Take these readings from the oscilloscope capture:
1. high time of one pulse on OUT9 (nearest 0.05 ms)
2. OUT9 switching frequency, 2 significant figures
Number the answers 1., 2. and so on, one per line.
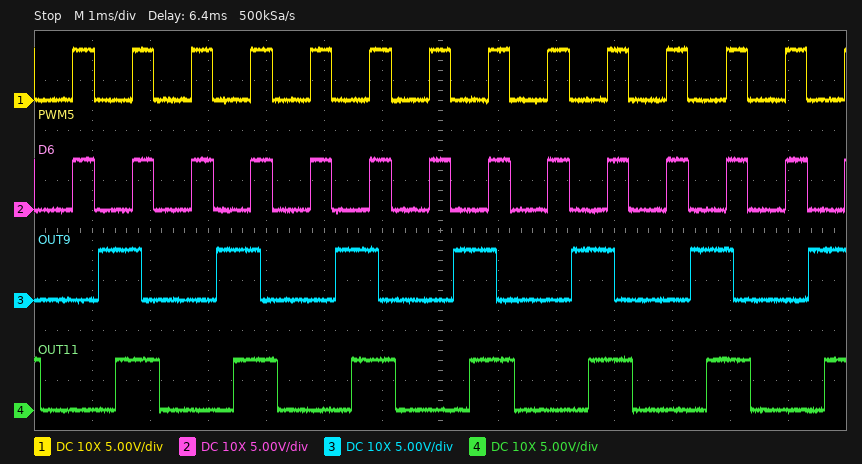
1. 0.75 ms
2. 490 Hz
